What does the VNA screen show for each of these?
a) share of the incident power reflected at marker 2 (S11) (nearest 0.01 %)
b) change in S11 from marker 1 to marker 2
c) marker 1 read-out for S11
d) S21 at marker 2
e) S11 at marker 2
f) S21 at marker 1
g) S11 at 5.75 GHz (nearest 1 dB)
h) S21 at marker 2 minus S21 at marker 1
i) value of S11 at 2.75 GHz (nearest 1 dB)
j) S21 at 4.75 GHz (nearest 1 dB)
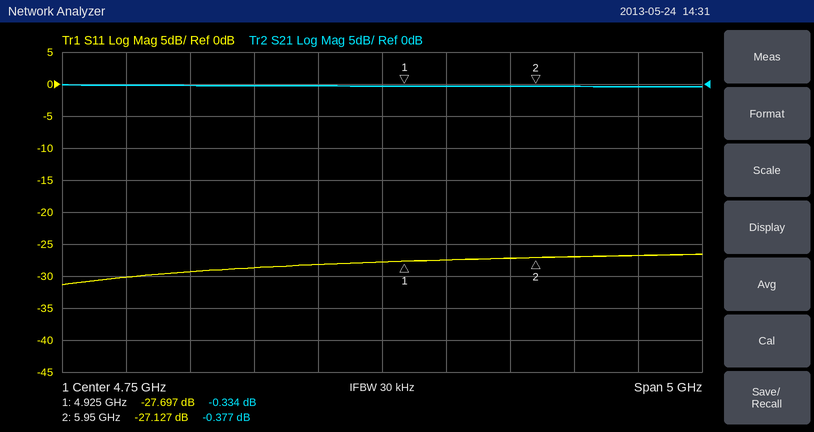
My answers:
0.19 %
0.570 dB
-27.697 dB
-0.377 dB
-27.127 dB
-0.334 dB
-27 dB
-0.043 dB
-30 dB
0 dB
